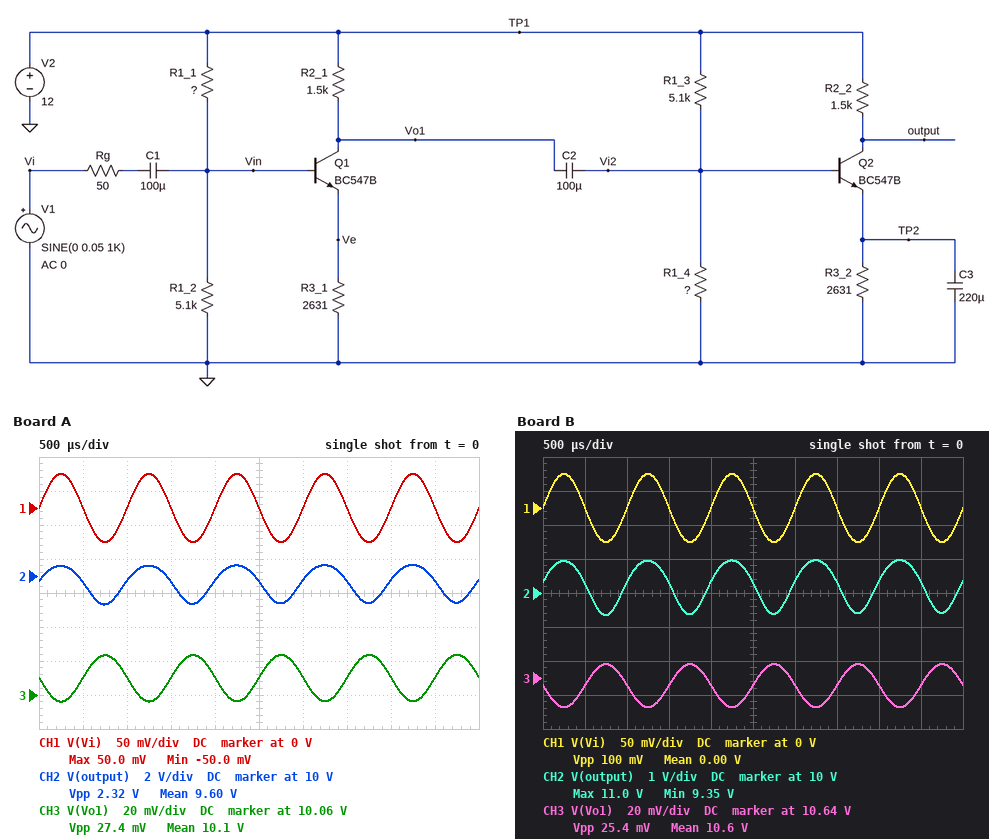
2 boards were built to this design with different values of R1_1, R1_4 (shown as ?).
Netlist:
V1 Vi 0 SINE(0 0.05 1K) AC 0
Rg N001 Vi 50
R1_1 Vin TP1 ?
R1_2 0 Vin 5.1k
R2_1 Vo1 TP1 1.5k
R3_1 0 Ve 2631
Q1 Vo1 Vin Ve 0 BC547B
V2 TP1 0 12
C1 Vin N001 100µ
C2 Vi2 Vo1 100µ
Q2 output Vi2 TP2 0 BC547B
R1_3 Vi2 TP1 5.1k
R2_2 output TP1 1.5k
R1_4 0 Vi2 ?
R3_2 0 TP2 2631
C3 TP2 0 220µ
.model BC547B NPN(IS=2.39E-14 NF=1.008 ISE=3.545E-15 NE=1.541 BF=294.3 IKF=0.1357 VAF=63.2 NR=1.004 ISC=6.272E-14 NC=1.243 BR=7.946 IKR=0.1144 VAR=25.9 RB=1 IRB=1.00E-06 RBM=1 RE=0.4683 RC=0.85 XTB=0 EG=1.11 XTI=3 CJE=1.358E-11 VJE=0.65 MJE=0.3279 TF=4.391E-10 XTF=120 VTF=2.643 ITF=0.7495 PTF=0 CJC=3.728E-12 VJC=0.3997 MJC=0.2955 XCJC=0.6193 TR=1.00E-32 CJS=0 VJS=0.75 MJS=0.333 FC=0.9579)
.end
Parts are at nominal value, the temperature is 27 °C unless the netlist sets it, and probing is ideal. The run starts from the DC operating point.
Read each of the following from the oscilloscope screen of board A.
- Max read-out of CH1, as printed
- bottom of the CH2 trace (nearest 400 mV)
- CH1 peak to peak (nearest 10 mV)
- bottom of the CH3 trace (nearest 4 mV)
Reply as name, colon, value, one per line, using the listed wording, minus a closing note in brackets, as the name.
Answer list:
Max read-out of CH1, as printed: 50.0 mV
bottom of the CH2 trace: 8.4 V
CH1 peak to peak: 100 mV
bottom of the CH3 trace: 10.056 V
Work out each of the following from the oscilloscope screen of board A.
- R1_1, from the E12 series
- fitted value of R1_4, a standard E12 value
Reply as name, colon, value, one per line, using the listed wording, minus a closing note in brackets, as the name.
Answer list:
R1_1, from the E12 series: 10 kΩ
fitted value of R1_4, a standard E12 value: 3.3 kΩ
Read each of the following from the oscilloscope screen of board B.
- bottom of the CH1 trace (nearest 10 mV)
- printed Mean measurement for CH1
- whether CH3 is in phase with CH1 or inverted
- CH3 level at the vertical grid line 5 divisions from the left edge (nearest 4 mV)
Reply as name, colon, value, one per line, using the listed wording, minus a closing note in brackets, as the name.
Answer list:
bottom of the CH1 trace: -50 mV
printed Mean measurement for CH1: 0.00 V
whether CH3 is in phase with CH1 or inverted: inverted
CH3 level at the vertical grid line 5 divisions from the left edge: 10.636 V
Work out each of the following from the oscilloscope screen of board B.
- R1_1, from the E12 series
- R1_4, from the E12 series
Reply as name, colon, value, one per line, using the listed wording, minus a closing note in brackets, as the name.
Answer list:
R1_1, from the E12 series: 15 kΩ
R1_4, from the E12 series: 2.2 kΩ
